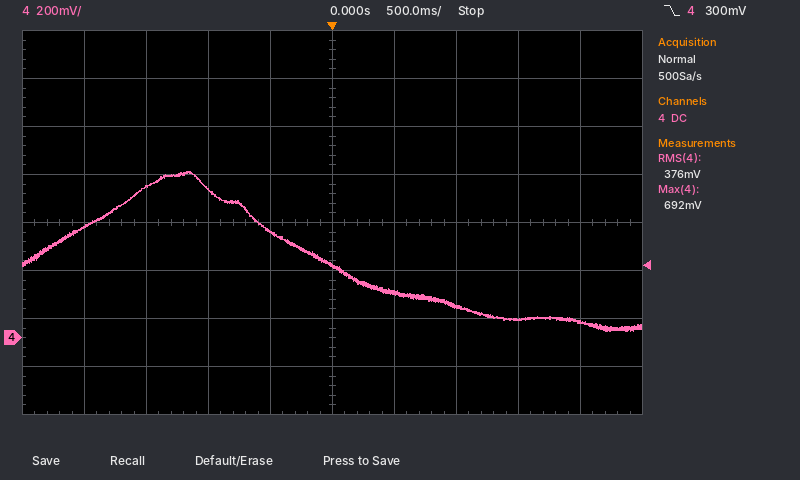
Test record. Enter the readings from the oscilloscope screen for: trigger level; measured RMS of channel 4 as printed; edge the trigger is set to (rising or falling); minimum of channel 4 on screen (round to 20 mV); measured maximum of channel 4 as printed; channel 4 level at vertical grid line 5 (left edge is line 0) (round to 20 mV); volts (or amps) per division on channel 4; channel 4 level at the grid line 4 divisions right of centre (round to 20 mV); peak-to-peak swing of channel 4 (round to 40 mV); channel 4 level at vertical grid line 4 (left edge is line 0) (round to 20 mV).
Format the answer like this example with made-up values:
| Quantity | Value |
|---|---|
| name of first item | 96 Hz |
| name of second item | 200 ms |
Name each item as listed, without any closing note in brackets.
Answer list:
| Quantity | Value |
|---|---|
| trigger level | 300 mV |
| measured RMS of channel 4 as printed | 376 mV |
| edge the trigger is set to | falling |
| minimum of channel 4 on screen | 20 mV |
| measured maximum of channel 4 as printed | 692 mV |
| channel 4 level at vertical grid line 5 (left edge is line 0) | 300 mV |
| volts (or amps) per division on channel 4 | 200 mV |
| channel 4 level at the grid line 4 divisions right of centre | 60 mV |
| peak-to-peak swing of channel 4 | 680 mV |
| channel 4 level at vertical grid line 4 (left edge is line 0) | 440 mV |
